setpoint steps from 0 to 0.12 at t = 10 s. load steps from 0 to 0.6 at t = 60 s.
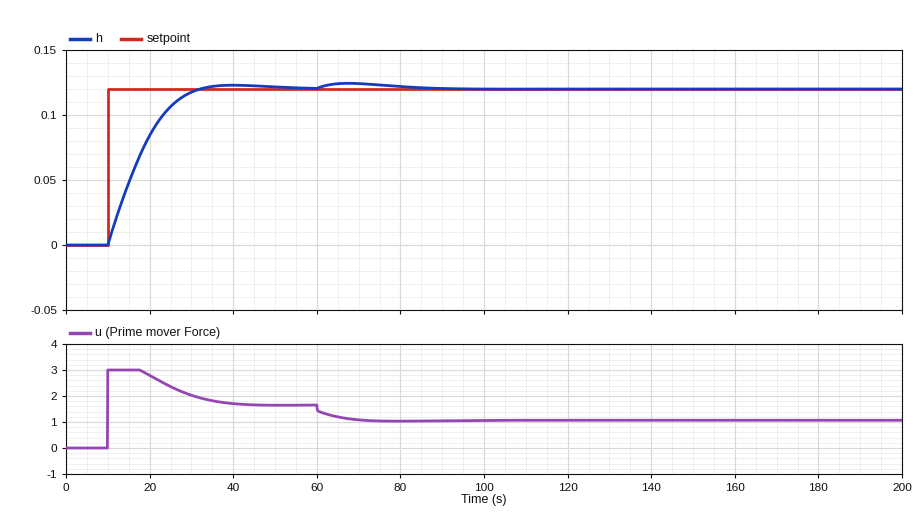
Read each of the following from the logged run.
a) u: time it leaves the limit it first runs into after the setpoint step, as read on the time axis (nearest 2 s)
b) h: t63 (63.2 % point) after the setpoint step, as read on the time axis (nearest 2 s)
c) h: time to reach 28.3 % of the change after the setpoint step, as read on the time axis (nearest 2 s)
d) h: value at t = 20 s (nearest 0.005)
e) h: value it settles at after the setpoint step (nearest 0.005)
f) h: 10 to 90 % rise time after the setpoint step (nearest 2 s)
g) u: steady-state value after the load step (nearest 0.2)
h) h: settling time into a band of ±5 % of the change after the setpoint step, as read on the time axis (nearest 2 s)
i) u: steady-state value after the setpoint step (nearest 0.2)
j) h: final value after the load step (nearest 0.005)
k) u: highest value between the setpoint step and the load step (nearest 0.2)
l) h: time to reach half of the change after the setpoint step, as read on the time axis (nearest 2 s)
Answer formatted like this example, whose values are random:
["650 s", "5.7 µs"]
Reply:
["18 s", "18 s", "14 s", "0.085", "0.120", "14 s", "1.0", "28 s", "1.6", "0.120", "3.0", "16 s"]
